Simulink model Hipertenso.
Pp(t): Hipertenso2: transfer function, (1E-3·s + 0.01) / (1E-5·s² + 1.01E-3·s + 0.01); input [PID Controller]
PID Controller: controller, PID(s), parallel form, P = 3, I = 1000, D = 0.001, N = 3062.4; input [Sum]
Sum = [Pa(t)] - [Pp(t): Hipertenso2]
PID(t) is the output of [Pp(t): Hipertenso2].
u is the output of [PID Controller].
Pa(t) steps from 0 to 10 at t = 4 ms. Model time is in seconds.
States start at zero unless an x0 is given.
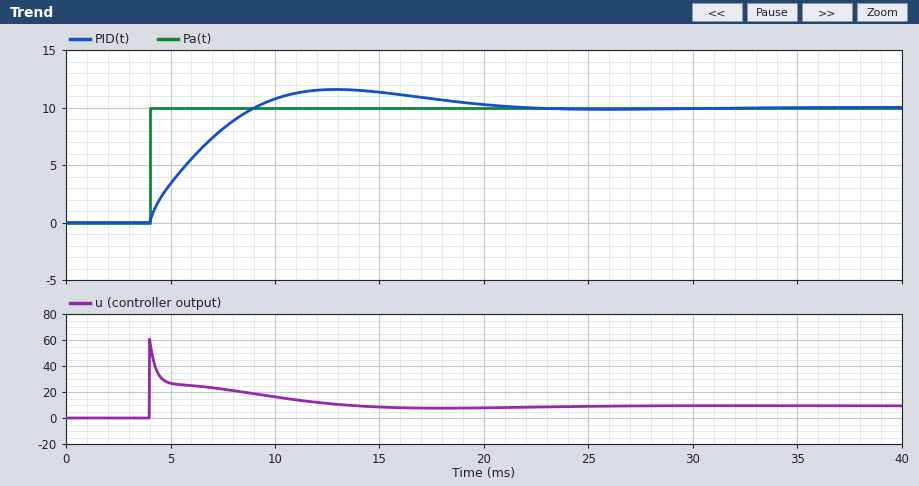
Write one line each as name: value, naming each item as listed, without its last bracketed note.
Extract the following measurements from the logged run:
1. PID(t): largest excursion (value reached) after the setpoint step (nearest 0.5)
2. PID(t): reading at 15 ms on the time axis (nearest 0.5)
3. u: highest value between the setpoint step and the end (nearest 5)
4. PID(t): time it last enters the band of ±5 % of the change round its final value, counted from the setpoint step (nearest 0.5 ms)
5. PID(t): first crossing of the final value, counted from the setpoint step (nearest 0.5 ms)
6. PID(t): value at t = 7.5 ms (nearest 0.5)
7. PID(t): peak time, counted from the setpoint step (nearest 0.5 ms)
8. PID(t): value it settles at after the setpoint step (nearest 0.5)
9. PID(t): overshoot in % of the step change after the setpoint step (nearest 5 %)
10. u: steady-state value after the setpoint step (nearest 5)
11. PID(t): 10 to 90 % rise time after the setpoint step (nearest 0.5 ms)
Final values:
PID(t): largest excursion (value reached) after the setpoint step: 11.5
PID(t): reading at 15 ms on the time axis: 11.5
u: highest value between the setpoint step and the end: 60
PID(t): time it last enters the band of ±5 % of the change round its final value, counted from the setpoint step: 14.5 ms
PID(t): first crossing of the final value, counted from the setpoint step: 5.0 ms
PID(t): value at t = 7.5 ms: 8.0
PID(t): peak time, counted from the setpoint step: 9.0 ms
PID(t): value it settles at after the setpoint step: 10.0
PID(t): overshoot in % of the step change after the setpoint step: 15 %
u: steady-state value after the setpoint step: 10
PID(t): 10 to 90 % rise time after the setpoint step: 4.0 ms
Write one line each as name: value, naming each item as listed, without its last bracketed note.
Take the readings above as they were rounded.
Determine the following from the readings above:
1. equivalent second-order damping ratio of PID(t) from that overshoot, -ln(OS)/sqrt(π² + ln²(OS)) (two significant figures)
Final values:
equivalent second-order damping ratio of PID(t) from that overshoot, -ln(OS)/sqrt(π² + ln²(OS)): 0.52
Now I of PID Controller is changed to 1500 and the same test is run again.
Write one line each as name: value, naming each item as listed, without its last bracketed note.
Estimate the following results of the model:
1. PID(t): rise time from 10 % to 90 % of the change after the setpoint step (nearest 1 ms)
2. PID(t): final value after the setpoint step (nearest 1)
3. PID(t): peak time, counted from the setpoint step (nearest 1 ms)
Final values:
PID(t): rise time from 10 % to 90 % of the change after the setpoint step: 3 ms
PID(t): final value after the setpoint step: 10
PID(t): peak time, counted from the setpoint step: 7 ms
